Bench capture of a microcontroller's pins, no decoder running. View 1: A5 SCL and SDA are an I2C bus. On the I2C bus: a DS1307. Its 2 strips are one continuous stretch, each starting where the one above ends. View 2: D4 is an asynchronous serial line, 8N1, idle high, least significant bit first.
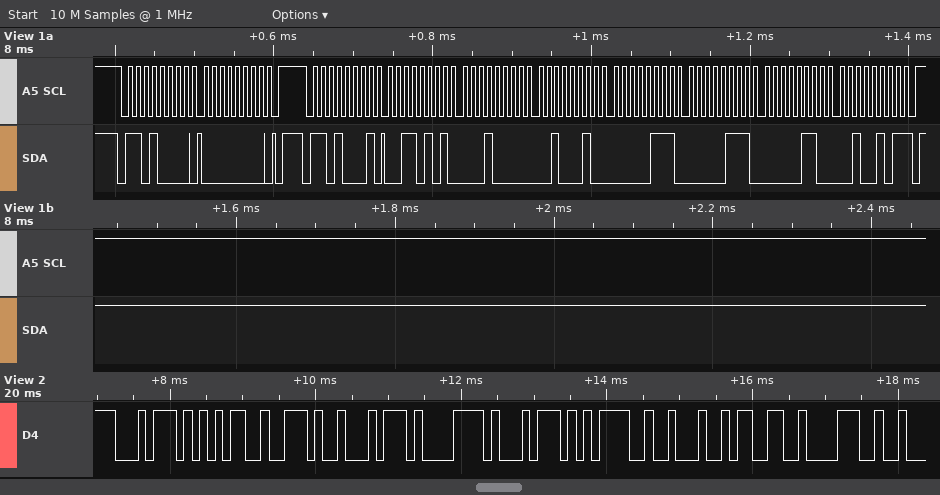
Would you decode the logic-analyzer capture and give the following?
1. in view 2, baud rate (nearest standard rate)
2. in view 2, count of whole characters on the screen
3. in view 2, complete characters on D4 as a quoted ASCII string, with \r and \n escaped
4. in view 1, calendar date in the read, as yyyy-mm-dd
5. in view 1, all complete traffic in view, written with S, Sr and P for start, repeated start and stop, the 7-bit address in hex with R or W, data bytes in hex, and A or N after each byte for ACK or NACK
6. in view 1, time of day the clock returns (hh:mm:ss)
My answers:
9600 baud
10
"t5.txt=\"38"
2025-06-07
S 68W A 00 A P S 68R A 35 A 10 A 22 A 07 A 07 A 06 A 25 N P
22:10:35
